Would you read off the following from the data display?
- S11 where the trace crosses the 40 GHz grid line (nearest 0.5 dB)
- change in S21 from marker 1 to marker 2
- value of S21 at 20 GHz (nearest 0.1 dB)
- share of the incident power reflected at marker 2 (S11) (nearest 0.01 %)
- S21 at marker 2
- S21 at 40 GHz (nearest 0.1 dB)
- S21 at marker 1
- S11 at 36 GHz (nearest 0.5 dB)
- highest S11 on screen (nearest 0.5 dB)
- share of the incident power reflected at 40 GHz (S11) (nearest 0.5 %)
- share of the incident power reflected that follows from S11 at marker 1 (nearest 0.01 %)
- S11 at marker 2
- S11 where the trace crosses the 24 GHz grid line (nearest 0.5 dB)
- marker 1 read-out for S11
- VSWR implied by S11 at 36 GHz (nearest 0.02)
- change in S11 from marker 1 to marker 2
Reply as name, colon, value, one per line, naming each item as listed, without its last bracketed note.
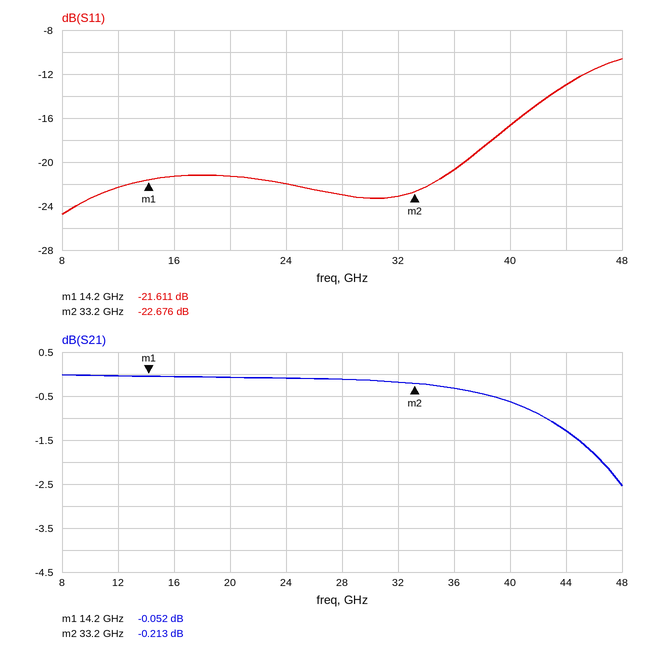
S11 where the trace crosses the 40 GHz grid line: -16.5 dB
change in S21 from marker 1 to marker 2: -0.161 dB
value of S21 at 20 GHz: -0.1 dB
share of the incident power reflected at marker 2 (S11): 0.54 %
S21 at marker 2: -0.213 dB
S21 at 40 GHz: -0.6 dB
S21 at marker 1: -0.052 dB
S11 at 36 GHz: -20.5 dB
highest S11 on screen: -10.5 dB
share of the incident power reflected at 40 GHz (S11): 2.0 %
share of the incident power reflected that follows from S11 at marker 1: 0.69 %
S11 at marker 2: -22.676 dB
S11 where the trace crosses the 24 GHz grid line: -22.0 dB
marker 1 read-out for S11: -21.611 dB
VSWR implied by S11 at 36 GHz: 1.20
change in S11 from marker 1 to marker 2: -1.065 dB
